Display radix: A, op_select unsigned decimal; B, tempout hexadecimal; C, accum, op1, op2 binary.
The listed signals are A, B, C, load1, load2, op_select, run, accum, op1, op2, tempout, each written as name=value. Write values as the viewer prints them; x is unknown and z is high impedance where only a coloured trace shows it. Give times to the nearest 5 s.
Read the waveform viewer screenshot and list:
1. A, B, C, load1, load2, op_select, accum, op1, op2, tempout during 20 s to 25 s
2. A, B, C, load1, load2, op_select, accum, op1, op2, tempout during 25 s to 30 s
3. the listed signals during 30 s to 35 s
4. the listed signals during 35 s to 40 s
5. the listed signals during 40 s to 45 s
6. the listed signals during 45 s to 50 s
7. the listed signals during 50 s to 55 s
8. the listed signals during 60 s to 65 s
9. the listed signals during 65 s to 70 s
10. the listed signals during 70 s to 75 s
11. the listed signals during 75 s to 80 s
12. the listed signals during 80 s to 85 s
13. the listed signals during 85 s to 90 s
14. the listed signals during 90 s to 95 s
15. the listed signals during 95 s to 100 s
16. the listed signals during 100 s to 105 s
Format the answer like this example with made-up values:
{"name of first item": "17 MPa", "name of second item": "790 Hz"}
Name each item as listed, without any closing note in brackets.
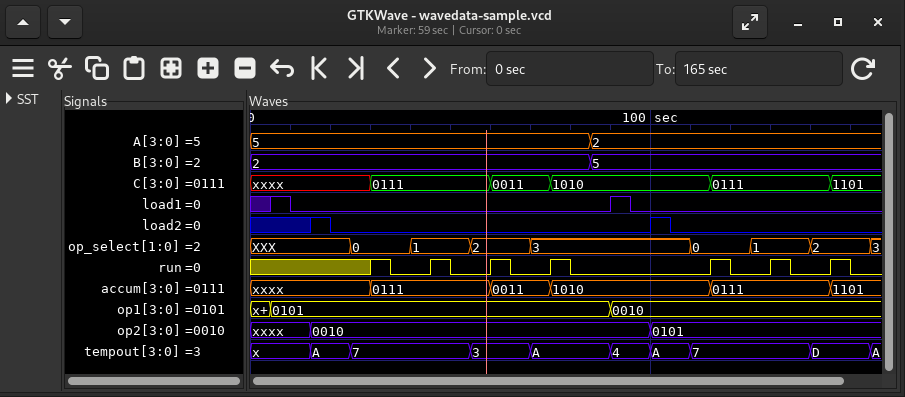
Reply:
{"A, B, C, load1, load2, op_select, accum, op1, op2, tempout during 20 s to 25 s": "A=5, B=2, C=xxxx, load1=0, load2=0, op_select=XXX, accum=xxxx, op1=0101, op2=0010, tempout=A", "A, B, C, load1, load2, op_select, accum, op1, op2, tempout during 25 s to 30 s": "A=5, B=2, C=xxxx, load1=0, load2=0, op_select=0, accum=xxxx, op1=0101, op2=0010, tempout=7", "the listed signals during 30 s to 35 s": "A=5, B=2, C=0111, load1=0, load2=0, op_select=0, run=1, accum=0111, op1=0101, op2=0010, tempout=7", "the listed signals during 35 s to 40 s": "A=5, B=2, C=0111, load1=0, load2=0, op_select=0, run=0, accum=0111, op1=0101, op2=0010, tempout=7", "the listed signals during 40 s to 45 s": "A=5, B=2, C=0111, load1=0, load2=0, op_select=1, run=0, accum=0111, op1=0101, op2=0010, tempout=7", "the listed signals during 45 s to 50 s": "A=5, B=2, C=0111, load1=0, load2=0, op_select=1, run=1, accum=0111, op1=0101, op2=0010, tempout=7", "the listed signals during 50 s to 55 s": "A=5, B=2, C=0111, load1=0, load2=0, op_select=1, run=0, accum=0111, op1=0101, op2=0010, tempout=7", "the listed signals during 60 s to 65 s": "A=5, B=2, C=0011, load1=0, load2=0, op_select=2, run=1, accum=0011, op1=0101, op2=0010, tempout=3", "the listed signals during 65 s to 70 s": "A=5, B=2, C=0011, load1=0, load2=0, op_select=2, run=0, accum=0011, op1=0101, op2=0010, tempout=3", "the listed signals during 70 s to 75 s": "A=5, B=2, C=0011, load1=0, load2=0, op_select=3, run=0, accum=0011, op1=0101, op2=0010, tempout=A", "the listed signals during 75 s to 80 s": "A=5, B=2, C=1010, load1=0, load2=0, op_select=3, run=1, accum=1010, op1=0101, op2=0010, tempout=A", "the listed signals during 80 s to 85 s": "A=5, B=2, C=1010, load1=0, load2=0, op_select=3, run=0, accum=1010, op1=0101, op2=0010, tempout=A", "the listed signals during 85 s to 90 s": "A=2, B=5, C=1010, load1=0, load2=0, op_select=3, run=0, accum=1010, op1=0101, op2=0010, tempout=A", "the listed signals during 90 s to 95 s": "A=2, B=5, C=1010, load1=1, load2=0, op_select=3, run=0, accum=1010, op1=0010, op2=0010, tempout=4", "the listed signals during 95 s to 100 s": "A=2, B=5, C=1010, load1=0, load2=0, op_select=3, run=0, accum=1010, op1=0010, op2=0010, tempout=4", "the listed signals during 100 s to 105 s": "A=2, B=5, C=1010, load1=0, load2=1, op_select=3, run=0, accum=1010, op1=0010, op2=0101, tempout=A"}
